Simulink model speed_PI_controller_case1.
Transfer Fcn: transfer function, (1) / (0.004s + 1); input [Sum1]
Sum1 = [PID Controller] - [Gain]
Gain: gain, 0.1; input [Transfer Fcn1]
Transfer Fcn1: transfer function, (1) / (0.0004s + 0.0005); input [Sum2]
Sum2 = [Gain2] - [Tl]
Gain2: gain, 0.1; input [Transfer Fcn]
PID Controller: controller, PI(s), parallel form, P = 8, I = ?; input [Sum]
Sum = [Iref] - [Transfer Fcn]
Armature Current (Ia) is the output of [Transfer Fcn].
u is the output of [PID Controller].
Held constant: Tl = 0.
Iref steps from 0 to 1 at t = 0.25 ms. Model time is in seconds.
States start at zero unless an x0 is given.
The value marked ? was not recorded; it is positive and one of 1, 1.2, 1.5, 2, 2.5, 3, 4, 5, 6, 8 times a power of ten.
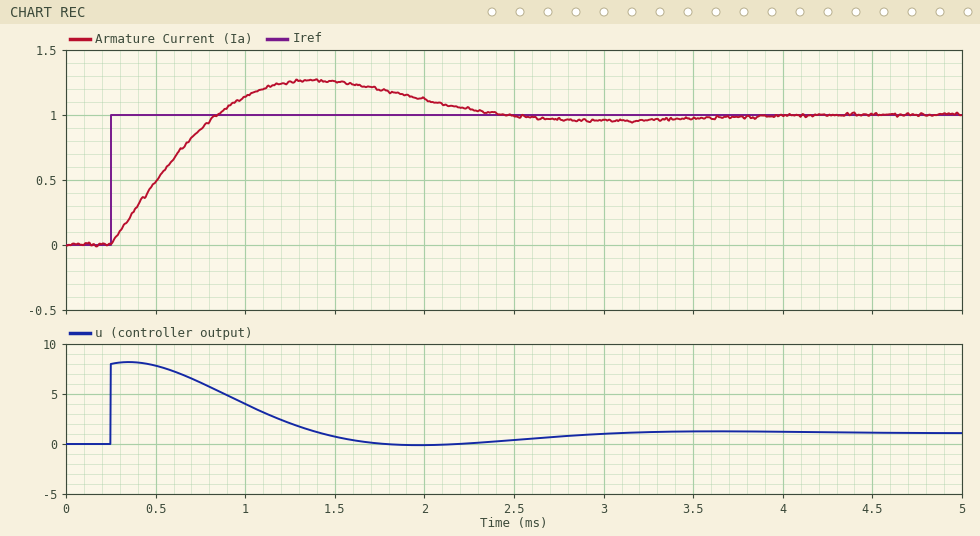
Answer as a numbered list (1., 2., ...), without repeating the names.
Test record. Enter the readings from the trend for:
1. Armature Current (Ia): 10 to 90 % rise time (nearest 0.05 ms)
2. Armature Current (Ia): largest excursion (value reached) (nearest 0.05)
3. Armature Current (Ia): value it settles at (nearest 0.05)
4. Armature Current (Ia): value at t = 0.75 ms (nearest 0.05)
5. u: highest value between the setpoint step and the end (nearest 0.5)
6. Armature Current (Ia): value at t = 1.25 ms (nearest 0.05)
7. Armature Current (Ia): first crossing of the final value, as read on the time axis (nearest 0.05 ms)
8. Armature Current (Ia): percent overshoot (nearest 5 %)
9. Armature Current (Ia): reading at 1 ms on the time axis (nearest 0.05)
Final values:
1. 0.45 ms
2. 1.25
3. 1.00
4. 0.90
5. 8.0
6. 1.25
7. 0.85 ms
8. 25 %
9. 1.15
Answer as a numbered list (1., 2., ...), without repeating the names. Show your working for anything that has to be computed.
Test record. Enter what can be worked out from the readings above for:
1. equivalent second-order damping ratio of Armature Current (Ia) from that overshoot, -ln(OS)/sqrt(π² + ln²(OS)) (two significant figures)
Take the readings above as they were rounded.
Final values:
1. ln(0.25) = -1.386; 1.386 / sqrt(9.870 + 1.922) = 0.40
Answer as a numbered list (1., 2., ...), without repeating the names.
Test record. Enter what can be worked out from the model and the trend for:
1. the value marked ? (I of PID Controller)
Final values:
1. 20000
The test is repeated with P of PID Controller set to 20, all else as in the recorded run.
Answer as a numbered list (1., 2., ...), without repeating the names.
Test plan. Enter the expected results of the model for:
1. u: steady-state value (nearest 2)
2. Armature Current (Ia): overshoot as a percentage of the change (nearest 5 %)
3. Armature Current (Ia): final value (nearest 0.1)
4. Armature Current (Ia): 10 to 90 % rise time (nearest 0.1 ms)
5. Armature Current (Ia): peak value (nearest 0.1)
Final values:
1. 2
2. 10 %
3. 1.0
4. 0.3 ms
5. 1.1
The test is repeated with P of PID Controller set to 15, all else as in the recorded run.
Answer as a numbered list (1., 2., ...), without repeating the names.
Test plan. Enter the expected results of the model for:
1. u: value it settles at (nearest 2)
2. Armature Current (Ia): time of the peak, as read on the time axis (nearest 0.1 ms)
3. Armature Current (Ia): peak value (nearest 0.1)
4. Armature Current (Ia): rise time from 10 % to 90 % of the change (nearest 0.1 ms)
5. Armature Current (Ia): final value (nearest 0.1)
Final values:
1. 2
2. 1.2 ms
3. 1.1
4. 0.4 ms
5. 1.0
